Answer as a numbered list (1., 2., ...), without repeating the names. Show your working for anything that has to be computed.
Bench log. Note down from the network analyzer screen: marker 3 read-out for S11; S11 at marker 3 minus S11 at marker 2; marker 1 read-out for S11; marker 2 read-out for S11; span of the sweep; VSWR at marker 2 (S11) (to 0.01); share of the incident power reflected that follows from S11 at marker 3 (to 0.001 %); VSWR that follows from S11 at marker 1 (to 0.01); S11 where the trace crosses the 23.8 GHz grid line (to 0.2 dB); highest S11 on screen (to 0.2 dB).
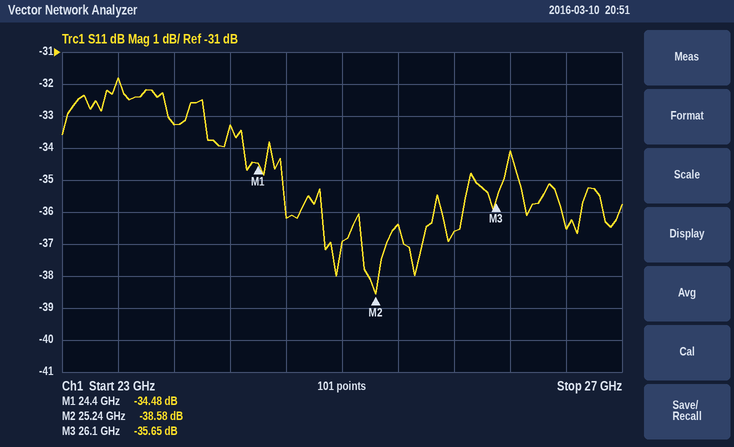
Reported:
1. -35.65 dB
2. -35.65 − (-38.58) = 2.93 dB
3. -34.48 dB
4. -38.58 dB
5. 4 GHz
6. (1 + 0.0118)/(1 − 0.0118) ≈ 1.02
7. 10^(-35.65/10) ≈ 0.027 %
8. (1 + 0.0189)/(1 − 0.0189) ≈ 1.04
9. -33.2 dB
10. -31.8 dB
